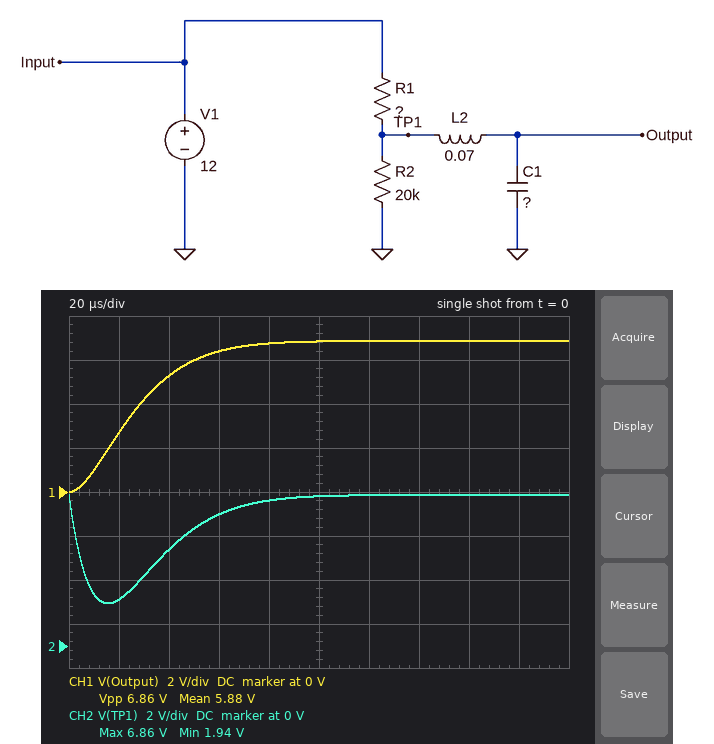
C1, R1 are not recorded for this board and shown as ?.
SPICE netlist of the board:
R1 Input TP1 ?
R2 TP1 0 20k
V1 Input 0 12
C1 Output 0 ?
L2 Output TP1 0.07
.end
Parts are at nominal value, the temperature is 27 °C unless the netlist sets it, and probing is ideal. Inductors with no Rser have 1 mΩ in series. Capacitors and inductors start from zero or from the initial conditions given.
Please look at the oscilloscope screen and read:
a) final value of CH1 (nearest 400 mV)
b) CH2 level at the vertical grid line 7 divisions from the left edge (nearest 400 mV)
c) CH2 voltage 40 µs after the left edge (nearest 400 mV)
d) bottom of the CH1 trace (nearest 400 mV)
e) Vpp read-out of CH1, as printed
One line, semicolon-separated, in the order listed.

6.8 V; 6.8 V; 4.4 V; 0 V; 6.86 V
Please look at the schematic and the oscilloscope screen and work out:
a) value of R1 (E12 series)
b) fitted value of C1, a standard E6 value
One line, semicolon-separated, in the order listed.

15 kΩ; 3.3 nF
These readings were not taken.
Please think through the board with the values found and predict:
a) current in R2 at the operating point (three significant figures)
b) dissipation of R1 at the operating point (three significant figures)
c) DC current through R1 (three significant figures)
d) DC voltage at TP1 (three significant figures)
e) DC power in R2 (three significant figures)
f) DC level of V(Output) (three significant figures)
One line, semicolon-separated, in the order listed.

343 µA; 1.76 mW; 343 µA; 6.86 V; 2.35 mW; 6.86 V
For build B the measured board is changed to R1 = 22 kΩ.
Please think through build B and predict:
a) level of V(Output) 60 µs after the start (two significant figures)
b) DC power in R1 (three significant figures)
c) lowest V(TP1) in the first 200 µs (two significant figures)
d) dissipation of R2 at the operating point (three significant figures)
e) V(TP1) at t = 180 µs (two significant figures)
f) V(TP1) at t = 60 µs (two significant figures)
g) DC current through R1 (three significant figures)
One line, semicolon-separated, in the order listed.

4.9 V; 1.80 mW; 1.3 V; 1.63 mW; 5.7 V; 4.6 V; 286 µA
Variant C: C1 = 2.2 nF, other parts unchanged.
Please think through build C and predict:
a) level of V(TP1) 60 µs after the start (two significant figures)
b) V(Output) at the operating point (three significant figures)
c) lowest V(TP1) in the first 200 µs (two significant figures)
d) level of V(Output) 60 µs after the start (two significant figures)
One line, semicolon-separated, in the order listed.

6.9 V; 6.86 V; 2.3 V; 7.0 V
